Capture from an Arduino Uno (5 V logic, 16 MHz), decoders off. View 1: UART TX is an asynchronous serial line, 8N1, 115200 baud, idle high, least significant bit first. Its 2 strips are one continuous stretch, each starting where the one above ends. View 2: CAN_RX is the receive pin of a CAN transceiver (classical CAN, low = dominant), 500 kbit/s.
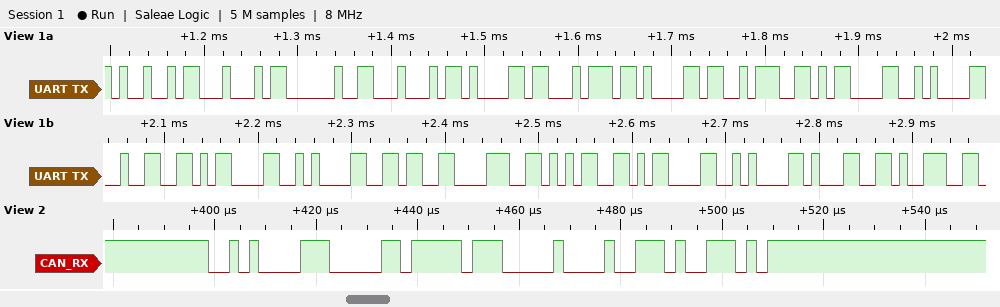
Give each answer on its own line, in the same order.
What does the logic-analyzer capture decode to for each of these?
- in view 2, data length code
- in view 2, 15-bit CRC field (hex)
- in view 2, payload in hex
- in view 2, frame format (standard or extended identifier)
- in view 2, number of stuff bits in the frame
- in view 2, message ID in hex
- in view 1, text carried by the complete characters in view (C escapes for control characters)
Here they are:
2
0x274E
FF 00
standard
3
0x287
"ID Data:\r\n2\r\n685\r\n19"
